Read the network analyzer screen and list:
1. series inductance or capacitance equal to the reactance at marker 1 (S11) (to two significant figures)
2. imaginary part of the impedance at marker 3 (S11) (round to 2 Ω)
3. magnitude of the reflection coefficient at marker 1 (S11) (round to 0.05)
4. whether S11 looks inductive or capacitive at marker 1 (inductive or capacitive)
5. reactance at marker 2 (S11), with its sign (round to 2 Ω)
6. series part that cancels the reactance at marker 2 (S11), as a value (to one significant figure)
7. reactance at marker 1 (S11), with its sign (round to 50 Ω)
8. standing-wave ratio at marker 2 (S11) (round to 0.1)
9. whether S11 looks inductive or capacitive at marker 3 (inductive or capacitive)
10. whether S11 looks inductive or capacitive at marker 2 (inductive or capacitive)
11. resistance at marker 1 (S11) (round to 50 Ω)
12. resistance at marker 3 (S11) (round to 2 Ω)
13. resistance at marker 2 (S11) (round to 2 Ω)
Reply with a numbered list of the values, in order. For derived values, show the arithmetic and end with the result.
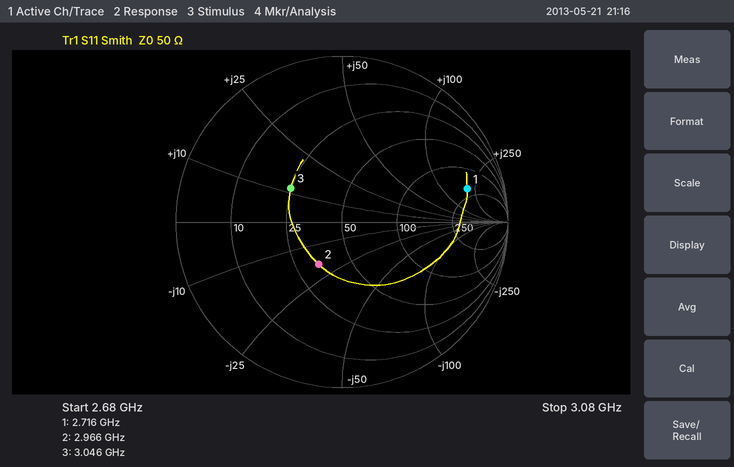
1. L = 200 Ω/(2π × 2.716 GHz) ≈ 12 nH
2. +12 Ω
3. 0.80
4. inductive
5. -18 Ω
6. L = 18 Ω/(2π × 2.966 GHz) ≈ 1.0 nH
7. +200 Ω
8. 1.8
9. inductive
10. capacitive
11. 200 Ω
12. 24 Ω
13. 34 Ω
